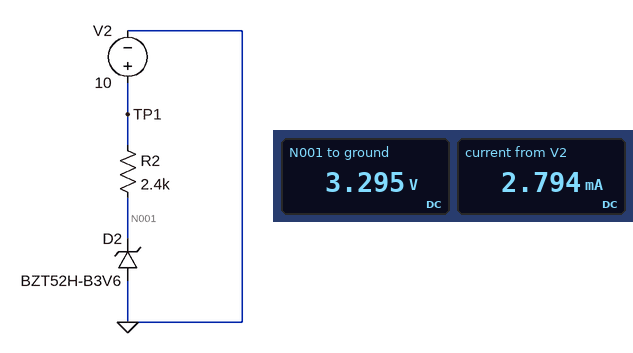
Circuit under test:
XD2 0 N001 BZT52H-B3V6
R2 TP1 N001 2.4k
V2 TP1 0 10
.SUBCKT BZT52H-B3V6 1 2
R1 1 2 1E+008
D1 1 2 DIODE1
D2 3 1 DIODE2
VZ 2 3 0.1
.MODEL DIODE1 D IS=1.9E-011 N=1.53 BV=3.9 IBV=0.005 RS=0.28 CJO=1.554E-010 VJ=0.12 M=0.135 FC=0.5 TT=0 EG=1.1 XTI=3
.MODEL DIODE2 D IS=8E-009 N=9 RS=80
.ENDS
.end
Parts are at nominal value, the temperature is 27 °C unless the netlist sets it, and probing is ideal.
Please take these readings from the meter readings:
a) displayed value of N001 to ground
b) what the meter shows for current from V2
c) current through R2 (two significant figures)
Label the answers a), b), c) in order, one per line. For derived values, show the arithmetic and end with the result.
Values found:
a) 3.295 V
b) 2.794 mA
c) (10 V - 3.295 V) / 2.4 kΩ = 2.8 mA
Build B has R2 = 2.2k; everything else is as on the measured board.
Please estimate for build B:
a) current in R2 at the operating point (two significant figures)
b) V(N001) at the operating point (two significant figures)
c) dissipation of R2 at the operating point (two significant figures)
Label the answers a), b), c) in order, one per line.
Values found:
a) 3.0 mA
b) 3.3 V
c) 20 mW
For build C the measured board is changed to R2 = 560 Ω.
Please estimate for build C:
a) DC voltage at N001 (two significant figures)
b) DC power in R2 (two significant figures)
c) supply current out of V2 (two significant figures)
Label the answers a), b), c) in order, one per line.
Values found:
a) 3.9 V
b) 67 mW
c) 11 mA
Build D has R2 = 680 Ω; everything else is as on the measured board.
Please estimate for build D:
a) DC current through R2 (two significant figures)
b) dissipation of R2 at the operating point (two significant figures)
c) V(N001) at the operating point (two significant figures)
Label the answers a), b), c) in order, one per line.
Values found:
a) 9.0 mA
b) 55 mW
c) 3.9 V
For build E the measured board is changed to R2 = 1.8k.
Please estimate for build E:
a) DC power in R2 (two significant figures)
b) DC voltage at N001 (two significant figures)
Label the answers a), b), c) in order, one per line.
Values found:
a) 24 mW
b) 3.4 V
